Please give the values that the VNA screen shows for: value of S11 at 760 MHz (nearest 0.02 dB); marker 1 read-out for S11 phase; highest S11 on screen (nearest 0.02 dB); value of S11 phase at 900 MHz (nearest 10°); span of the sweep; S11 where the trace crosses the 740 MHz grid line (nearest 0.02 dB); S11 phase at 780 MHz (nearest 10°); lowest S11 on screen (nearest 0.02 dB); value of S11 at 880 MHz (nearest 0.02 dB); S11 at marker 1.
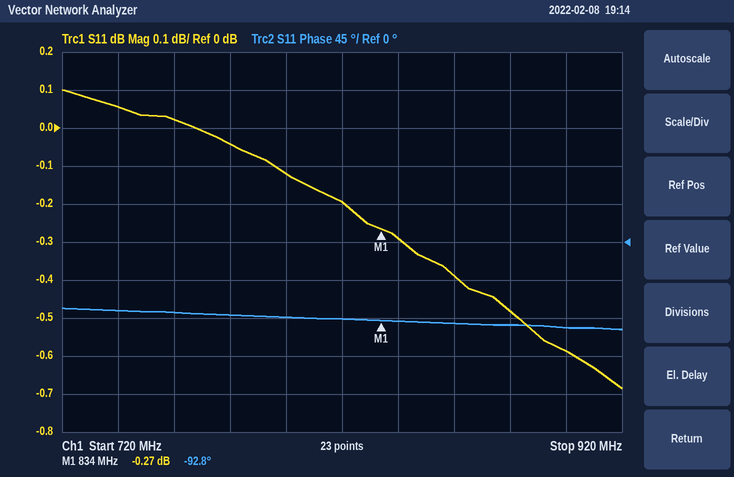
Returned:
0.02 dB
-92.8°
0.10 dB
-100°
200 MHz
0.06 dB
-90°
-0.68 dB
-0.48 dB
-0.27 dB
